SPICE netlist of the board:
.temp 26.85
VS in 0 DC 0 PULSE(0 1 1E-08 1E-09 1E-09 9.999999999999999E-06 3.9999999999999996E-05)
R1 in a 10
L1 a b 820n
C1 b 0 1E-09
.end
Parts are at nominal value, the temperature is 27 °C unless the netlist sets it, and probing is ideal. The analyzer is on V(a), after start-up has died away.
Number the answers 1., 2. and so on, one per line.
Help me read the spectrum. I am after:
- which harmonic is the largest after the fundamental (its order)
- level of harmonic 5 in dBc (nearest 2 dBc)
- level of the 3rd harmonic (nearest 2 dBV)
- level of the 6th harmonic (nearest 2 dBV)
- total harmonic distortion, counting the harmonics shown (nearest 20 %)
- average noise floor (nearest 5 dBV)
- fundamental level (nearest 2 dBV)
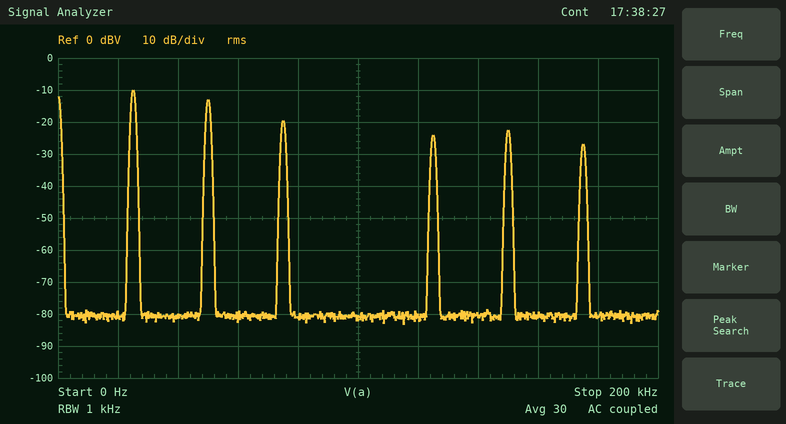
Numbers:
1. 2
2. -14 dBc
3. -20 dBV
4. -22 dBV
5. 80 %
6. -80 dBV
7. -10 dBV
